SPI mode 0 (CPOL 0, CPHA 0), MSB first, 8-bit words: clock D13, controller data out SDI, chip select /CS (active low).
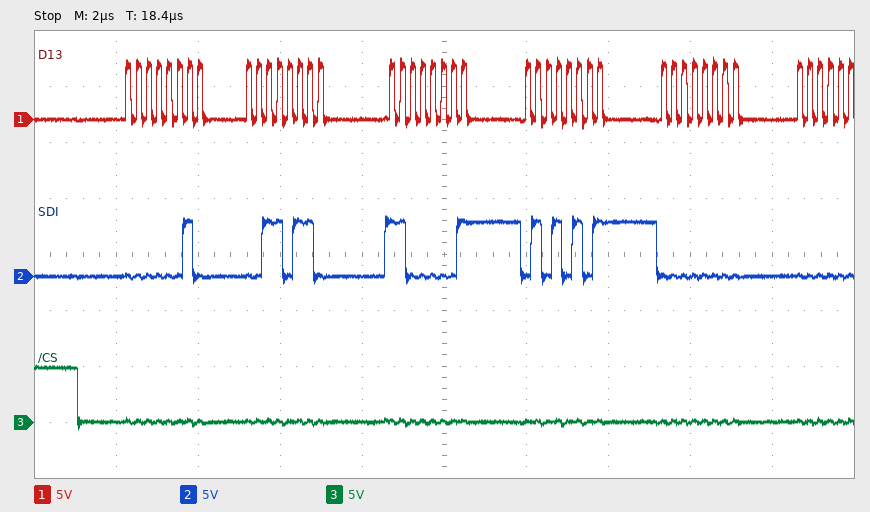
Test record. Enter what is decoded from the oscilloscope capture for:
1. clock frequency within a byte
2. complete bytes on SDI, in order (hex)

4 MHz
02 36 C1 55 00
